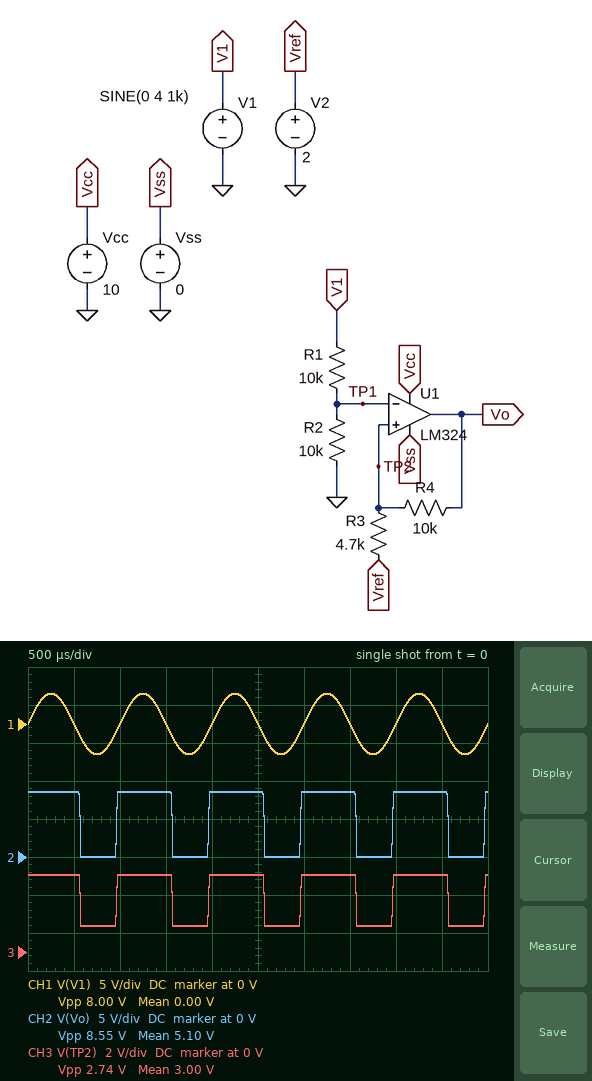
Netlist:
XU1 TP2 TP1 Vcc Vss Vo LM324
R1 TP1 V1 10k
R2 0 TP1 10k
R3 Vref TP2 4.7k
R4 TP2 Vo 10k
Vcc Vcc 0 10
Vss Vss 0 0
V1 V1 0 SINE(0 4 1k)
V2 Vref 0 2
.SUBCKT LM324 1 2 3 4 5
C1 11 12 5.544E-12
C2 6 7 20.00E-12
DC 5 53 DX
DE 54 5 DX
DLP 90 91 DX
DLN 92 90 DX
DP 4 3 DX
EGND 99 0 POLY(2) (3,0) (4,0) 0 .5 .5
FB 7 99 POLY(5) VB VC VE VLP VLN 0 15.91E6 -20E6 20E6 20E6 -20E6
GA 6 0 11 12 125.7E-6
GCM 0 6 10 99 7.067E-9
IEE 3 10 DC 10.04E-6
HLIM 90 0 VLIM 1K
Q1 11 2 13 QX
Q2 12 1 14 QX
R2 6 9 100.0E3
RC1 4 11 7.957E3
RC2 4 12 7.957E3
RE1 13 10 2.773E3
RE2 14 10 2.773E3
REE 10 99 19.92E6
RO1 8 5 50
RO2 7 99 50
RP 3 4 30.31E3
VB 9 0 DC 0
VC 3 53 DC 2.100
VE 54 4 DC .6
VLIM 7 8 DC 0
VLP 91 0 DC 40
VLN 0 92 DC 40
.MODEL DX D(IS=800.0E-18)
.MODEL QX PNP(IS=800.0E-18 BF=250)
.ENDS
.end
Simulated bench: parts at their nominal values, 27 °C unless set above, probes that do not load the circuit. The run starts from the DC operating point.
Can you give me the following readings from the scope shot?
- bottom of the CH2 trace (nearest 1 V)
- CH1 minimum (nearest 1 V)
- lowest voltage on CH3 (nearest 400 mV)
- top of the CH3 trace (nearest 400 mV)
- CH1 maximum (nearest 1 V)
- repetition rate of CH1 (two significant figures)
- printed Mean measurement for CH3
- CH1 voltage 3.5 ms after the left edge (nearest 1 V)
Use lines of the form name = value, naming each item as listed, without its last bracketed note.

bottom of the CH2 trace = 0 V
CH1 minimum = -4 V
lowest voltage on CH3 = 1.2 V
top of the CH3 trace = 4.0 V
CH1 maximum = 4 V
repetition rate of CH1 = 1.0 kHz
printed Mean measurement for CH3 = 3.00 V
CH1 voltage 3.5 ms after the left edge = 0 V
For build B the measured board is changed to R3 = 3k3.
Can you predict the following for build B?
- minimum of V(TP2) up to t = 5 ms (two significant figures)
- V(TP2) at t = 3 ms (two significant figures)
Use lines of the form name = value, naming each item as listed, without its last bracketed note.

minimum of V(TP2) up to t = 5 ms = 1.5 V
V(TP2) at t = 3 ms = 3.6 V
